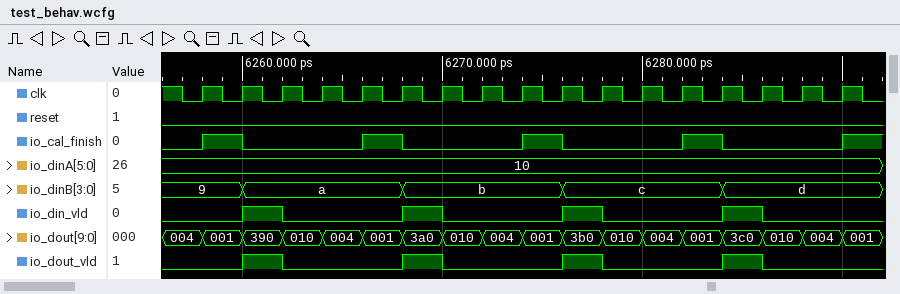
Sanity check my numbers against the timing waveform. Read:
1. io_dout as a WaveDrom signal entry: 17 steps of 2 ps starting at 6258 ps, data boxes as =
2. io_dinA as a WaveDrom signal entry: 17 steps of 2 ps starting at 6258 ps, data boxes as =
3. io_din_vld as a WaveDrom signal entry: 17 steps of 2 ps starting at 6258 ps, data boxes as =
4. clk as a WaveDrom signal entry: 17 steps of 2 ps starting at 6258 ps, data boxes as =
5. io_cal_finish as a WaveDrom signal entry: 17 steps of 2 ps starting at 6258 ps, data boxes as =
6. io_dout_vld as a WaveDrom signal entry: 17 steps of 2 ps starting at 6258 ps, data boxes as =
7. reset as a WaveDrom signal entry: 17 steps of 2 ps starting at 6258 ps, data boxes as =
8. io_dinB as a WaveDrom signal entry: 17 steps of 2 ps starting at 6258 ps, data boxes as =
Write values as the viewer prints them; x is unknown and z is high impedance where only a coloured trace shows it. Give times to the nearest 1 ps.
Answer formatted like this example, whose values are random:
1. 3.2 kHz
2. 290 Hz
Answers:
1. {name: 'io_dout', wave: '=================', data: '001 390 010 004 001 3a0 010 004 001 3b0 010 004 001 3c0 010 004 001'}
2. {name: 'io_dinA', wave: '=................', data: '10'}
3. {name: 'io_din_vld', wave: '010..10..10..10..'}
4. {name: 'clk', wave: 'p................'}
5. {name: 'io_cal_finish', wave: '10..10..10..10..1'}
6. {name: 'io_dout_vld', wave: '010..10..10..10..'}
7. {name: 'reset', wave: '0................'}
8. {name: 'io_dinB', wave: '==...=...=...=...', data: '9 a b c d'}
